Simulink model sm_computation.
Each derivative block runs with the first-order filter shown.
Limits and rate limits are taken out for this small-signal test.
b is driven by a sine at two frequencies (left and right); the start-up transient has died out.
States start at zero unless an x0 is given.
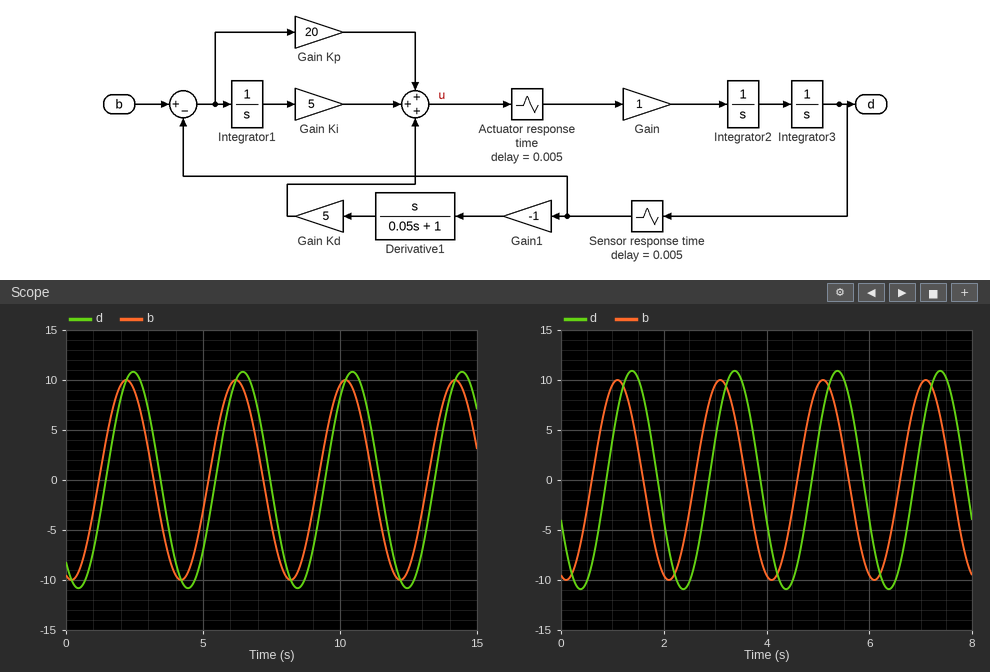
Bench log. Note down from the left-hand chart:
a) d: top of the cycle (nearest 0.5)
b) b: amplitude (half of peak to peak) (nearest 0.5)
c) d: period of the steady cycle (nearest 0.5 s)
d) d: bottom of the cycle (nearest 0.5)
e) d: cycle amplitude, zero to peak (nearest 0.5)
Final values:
11.0
10.0
4.0 s
-11.0
11.0
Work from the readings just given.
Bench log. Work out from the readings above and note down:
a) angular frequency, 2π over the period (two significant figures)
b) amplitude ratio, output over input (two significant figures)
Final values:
1.6 rad/s
1.1
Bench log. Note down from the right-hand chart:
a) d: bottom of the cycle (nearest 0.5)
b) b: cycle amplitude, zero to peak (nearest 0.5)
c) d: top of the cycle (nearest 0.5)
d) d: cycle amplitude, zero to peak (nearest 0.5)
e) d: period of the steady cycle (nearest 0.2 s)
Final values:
-11.0
10.0
11.0
11.0
2.0 s
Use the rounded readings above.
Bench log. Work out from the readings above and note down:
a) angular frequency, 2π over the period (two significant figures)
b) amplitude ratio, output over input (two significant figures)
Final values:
3.1 rad/s
1.1
